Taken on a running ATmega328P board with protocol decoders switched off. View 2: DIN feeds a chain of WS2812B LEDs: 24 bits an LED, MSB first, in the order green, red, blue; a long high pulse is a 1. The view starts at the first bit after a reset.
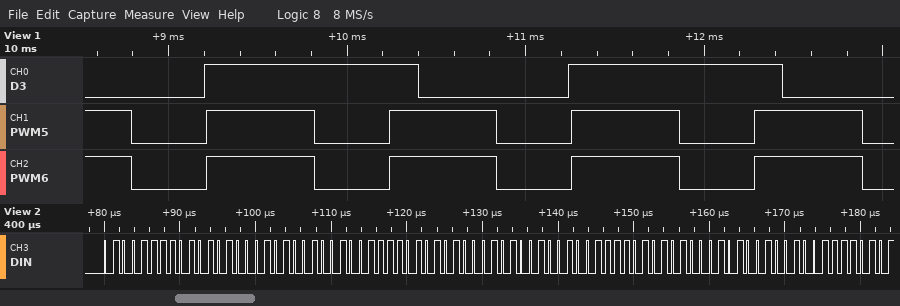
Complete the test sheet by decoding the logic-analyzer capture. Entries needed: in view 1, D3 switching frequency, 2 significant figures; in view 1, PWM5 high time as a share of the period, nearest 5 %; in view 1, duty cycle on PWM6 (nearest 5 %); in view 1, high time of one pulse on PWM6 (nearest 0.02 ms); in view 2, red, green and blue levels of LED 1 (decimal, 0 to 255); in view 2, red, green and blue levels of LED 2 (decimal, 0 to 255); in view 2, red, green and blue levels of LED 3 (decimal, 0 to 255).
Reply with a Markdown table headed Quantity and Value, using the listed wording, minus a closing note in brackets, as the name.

| Quantity | Value |
|---|---|
| in view 1, D3 switching frequency, 2 significant figures | 490 Hz |
| in view 1, PWM5 high time as a share of the period, nearest 5 % | 60 % |
| in view 1, duty cycle on PWM6 | 60 % |
| in view 1, high time of one pulse on PWM6 | 0.60 ms |
| in view 2, red, green and blue levels of LED 1 | 84, 79, 82 |
| in view 2, red, green and blue levels of LED 2 | 84, 79, 82 |
| in view 2, red, green and blue levels of LED 3 | 84, 79, 82 |
